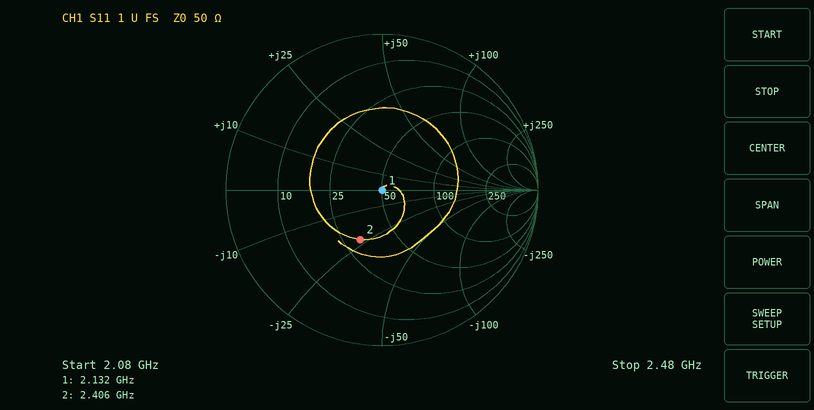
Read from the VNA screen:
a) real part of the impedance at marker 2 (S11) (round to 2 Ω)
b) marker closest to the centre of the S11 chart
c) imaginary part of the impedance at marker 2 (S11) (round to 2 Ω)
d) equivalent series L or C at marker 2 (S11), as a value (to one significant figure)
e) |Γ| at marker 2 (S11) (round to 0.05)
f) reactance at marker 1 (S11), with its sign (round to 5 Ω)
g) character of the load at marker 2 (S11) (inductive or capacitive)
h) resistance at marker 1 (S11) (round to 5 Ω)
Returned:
32 Ω
marker 1
-22 Ω
3 pF
0.35
0 Ω
capacitive
50 Ω
